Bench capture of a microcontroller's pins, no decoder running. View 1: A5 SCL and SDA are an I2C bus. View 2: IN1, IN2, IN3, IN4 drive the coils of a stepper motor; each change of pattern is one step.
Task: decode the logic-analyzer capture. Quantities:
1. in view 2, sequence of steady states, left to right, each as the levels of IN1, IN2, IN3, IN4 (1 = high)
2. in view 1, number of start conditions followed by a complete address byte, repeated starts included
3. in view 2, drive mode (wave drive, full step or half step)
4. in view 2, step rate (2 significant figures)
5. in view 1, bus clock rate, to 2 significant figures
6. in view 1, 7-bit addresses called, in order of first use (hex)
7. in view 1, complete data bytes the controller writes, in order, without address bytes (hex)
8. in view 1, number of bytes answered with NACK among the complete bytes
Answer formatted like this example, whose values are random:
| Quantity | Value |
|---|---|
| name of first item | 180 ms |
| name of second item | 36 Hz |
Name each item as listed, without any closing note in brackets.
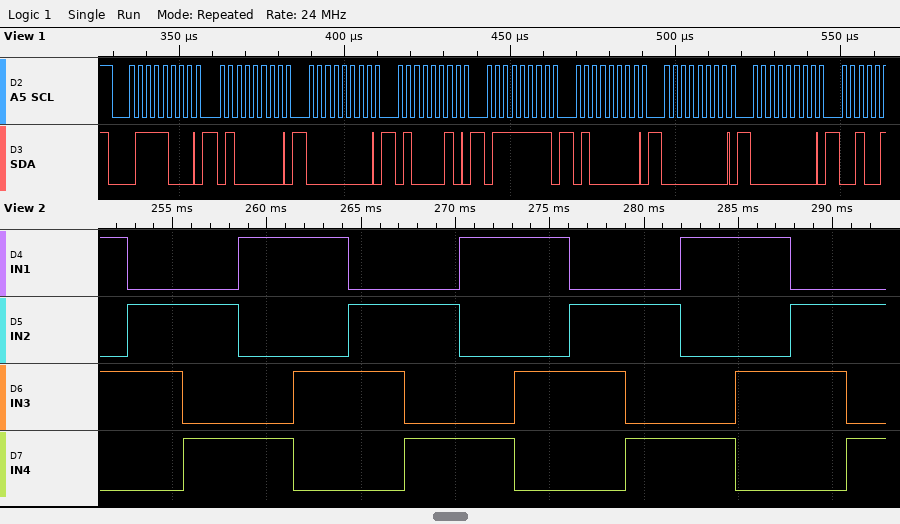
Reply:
| Quantity | Value |
|---|---|
| in view 2, sequence of steady states, left to right, each as the levels of IN1, IN2, IN3, IN4 | 1010 0110 0101 1001 1010 0110 0101 1001 1010 0110 0101 1001 1010 0110 0101 |
| in view 1, number of start conditions followed by a complete address byte, repeated starts included | 1 |
| in view 2, drive mode | full step |
| in view 2, step rate | 340 steps/s |
| in view 1, bus clock rate, to 2 significant figures | 400 kHz |
| in view 1, 7-bit addresses called, in order of first use | 0x3C |
| in view 1, complete data bytes the controller writes, in order, without address bytes | 40 00 42 7F 40 00 00 |
| in view 1, number of bytes answered with NACK among the complete bytes | 0 |
